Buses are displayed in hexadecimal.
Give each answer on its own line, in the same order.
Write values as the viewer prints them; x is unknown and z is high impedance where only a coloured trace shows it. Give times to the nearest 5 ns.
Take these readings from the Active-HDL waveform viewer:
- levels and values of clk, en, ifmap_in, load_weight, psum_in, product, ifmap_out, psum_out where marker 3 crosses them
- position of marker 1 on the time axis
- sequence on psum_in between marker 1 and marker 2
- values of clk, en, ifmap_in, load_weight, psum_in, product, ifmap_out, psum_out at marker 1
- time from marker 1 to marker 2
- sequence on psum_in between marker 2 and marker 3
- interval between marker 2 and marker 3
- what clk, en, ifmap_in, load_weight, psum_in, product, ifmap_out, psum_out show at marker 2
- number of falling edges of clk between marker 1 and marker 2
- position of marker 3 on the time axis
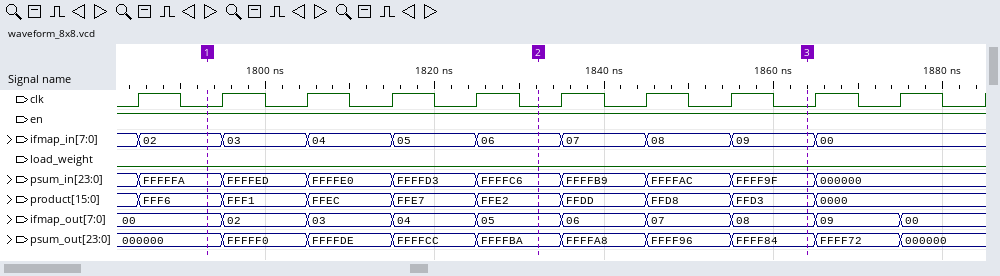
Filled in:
clk=0, en=1, ifmap_in=09, load_weight=0, psum_in=FFFF9F, product=FFD3, ifmap_out=08, psum_out=FFFF84
1795 ns
FFFFFA, FFFFED, FFFFE0, FFFFD3, FFFFC6
clk=0, en=1, ifmap_in=02, load_weight=0, psum_in=FFFFFA, product=FFF6, ifmap_out=00, psum_out=000000
40 ns
FFFFC6, FFFFB9, FFFFAC, FFFF9F
30 ns
clk=0, en=1, ifmap_in=06, load_weight=0, psum_in=FFFFC6, product=FFE2, ifmap_out=05, psum_out=FFFFBA
4
1865 ns
